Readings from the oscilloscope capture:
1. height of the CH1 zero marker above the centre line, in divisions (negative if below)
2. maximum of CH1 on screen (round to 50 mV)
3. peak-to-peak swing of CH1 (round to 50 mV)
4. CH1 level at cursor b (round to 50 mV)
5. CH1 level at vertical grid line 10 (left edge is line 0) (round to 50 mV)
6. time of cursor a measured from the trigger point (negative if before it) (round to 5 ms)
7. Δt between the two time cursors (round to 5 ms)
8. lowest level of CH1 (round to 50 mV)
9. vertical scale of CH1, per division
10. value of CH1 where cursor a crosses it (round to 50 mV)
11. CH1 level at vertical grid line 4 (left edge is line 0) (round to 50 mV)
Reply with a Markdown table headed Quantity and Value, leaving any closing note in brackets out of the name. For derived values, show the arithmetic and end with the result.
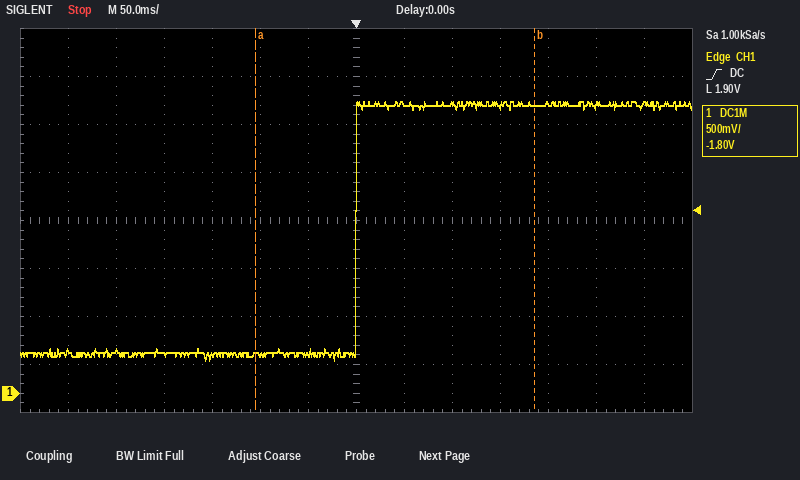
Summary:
| Quantity | Value |
|---|---|
| height of the CH1 zero marker above the centre line, in divisions | -3.6 div |
| maximum of CH1 on screen | 3.05 V |
| peak-to-peak swing of CH1 | 3.05 V − (350 mV) = 2.70 V |
| CH1 level at cursor b | 3.00 V |
| CH1 level at vertical grid line 10 (left edge is line 0) | 3.00 V |
| time of cursor a measured from the trigger point (negative if before it) | -105 ms |
| Δt between the two time cursors | 290 ms |
| lowest level of CH1 | 350 mV |
| vertical scale of CH1, per division | 500 mV |
| value of CH1 where cursor a crosses it | 400 mV |
| CH1 level at vertical grid line 4 (left edge is line 0) | 400 mV |
